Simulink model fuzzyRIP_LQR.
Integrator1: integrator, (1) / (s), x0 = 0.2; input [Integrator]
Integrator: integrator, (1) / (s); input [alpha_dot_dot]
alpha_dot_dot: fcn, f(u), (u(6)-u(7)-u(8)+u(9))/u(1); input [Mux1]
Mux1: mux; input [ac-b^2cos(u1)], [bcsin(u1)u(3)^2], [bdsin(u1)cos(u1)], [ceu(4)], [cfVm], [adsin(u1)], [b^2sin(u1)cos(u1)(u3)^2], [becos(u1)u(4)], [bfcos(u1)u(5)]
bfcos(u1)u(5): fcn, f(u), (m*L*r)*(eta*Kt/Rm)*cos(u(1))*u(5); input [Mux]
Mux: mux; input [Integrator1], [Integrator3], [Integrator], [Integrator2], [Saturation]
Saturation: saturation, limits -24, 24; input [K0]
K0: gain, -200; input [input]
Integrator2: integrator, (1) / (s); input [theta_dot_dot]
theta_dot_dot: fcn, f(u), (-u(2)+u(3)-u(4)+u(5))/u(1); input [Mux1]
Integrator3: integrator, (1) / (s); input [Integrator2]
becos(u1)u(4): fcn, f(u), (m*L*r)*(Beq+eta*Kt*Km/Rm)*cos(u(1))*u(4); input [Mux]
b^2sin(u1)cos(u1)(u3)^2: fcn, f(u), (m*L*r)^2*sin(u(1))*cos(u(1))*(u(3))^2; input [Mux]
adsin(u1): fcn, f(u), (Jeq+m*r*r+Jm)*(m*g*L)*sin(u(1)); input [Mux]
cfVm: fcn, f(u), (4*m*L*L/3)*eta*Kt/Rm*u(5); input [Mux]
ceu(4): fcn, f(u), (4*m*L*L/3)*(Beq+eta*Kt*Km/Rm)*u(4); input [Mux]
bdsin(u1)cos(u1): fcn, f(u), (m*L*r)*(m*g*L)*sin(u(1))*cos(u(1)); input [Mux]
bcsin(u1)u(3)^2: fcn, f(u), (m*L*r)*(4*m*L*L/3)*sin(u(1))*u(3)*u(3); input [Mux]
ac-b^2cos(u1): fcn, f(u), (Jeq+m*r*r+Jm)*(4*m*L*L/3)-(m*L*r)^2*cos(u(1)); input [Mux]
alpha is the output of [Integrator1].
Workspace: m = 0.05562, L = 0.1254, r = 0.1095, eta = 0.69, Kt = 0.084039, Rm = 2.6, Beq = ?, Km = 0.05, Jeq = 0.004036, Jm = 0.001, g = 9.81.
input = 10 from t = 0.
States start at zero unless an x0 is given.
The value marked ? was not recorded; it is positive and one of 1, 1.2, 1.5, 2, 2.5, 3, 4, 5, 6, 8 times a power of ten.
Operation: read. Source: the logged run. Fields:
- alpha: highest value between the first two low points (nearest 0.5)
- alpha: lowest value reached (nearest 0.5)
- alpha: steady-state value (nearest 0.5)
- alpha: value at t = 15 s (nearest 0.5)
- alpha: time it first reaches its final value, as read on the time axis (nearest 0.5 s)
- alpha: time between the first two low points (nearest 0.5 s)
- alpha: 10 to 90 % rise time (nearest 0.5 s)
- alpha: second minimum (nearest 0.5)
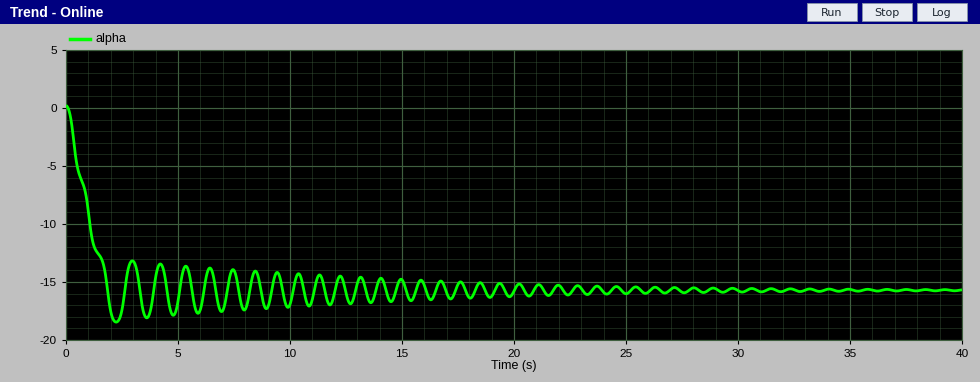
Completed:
-13.0
-18.5
-15.5
-15.0
2.0 s
1.5 s
1.5 s
-18.0
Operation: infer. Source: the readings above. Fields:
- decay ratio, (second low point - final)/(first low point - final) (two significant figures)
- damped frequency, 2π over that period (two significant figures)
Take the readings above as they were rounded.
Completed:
0.83
4.2 rad/s
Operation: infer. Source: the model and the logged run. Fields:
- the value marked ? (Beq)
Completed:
0.02
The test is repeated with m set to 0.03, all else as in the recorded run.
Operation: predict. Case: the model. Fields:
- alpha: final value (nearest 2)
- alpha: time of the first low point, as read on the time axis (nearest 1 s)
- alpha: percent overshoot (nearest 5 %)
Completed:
-22
3 s
15 %
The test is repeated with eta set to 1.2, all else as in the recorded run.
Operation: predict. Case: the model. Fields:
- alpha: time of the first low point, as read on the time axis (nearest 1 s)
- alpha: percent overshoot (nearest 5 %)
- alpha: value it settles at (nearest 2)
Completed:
3 s
15 %
-22
